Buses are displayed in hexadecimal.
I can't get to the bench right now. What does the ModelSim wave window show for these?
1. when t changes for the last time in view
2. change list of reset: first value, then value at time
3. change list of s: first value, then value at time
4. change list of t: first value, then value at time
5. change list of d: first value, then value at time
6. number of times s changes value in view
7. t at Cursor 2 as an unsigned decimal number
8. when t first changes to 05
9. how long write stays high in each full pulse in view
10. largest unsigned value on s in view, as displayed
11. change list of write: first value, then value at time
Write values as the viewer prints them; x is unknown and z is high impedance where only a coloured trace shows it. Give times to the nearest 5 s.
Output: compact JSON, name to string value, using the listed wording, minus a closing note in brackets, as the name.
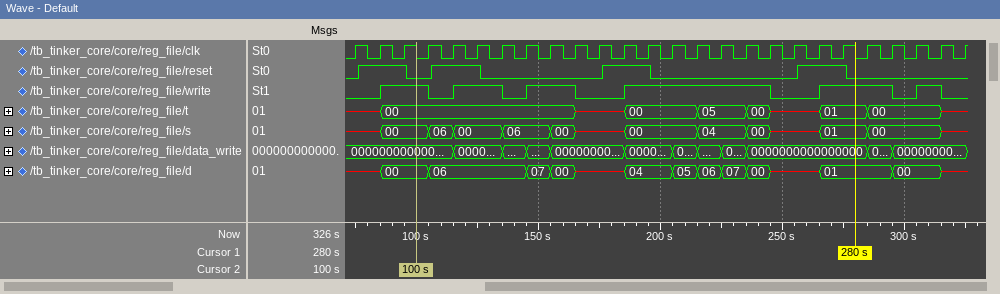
{"when t changes for the last time in view": "315 s", "change list of reset: first value, then value at time": "0, 1 at 75 s, 0 at 95 s, 1 at 105 s, 0 at 125 s, 1 at 175 s, 0 at 195 s, 1 at 255 s, 0 at 275 s", "change list of s: first value, then value at time": "x, 00 at 85 s, 06 at 105 s, 00 at 115 s, 06 at 135 s, 00 at 155 s, x at 165 s, 00 at 185 s, 04 at 215 s, 00 at 235 s, x at 245 s, 01 at 265 s, 00 at 285 s, x at 315 s", "change list of t: first value, then value at time": "x, 00 at 85 s, x at 165 s, 00 at 185 s, 05 at 215 s, 00 at 235 s, x at 245 s, 01 at 265 s, 00 at 285 s, x at 315 s", "change list of d: first value, then value at time": "x, 00 at 85 s, 06 at 105 s, 07 at 145 s, 00 at 155 s, x at 165 s, 04 at 185 s, 05 at 205 s, 06 at 215 s, 07 at 225 s, 00 at 235 s, x at 245 s, 01 at 265 s, 00 at 295 s, x at 315 s", "number of times s changes value in view": "13", "t at Cursor 2 as an unsigned decimal number": "0", "when t first changes to 05": "215 s", "how long write stays high in each full pulse in view": "20 s, 20 s, 20 s, 60 s, 30 s, 10 s", "largest unsigned value on s in view, as displayed": "06", "change list of write: first value, then value at time": "0, 1 at 85 s, 0 at 105 s, 1 at 115 s, 0 at 135 s, 1 at 145 s, 0 at 165 s, 1 at 185 s, 0 at 245 s, 1 at 265 s, 0 at 295 s, 1 at 305 s, 0 at 315 s"}
